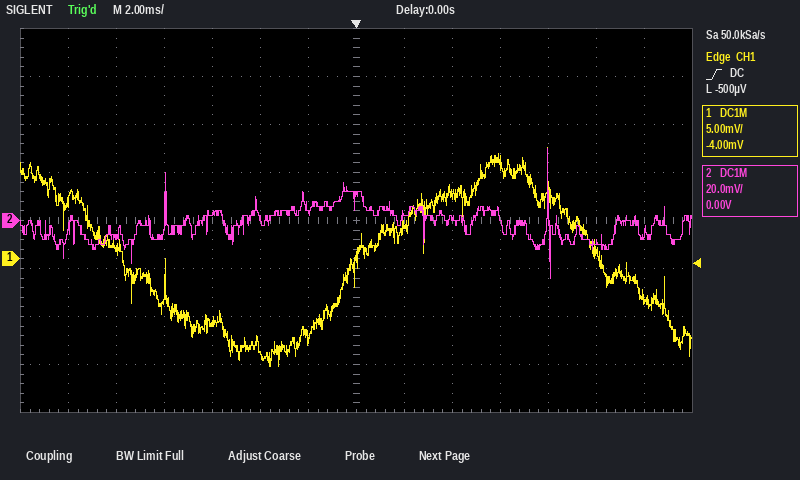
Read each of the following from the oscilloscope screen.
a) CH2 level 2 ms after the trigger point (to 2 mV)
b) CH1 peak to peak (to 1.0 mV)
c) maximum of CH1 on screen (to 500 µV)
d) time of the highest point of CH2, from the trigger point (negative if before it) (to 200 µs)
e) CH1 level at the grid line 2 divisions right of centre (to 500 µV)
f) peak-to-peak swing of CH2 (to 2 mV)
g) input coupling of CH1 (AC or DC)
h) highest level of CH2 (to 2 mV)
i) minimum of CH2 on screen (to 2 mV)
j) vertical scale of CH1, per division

2 mV
23.0 mV
11.5 mV
+8.0 ms
6.5 mV
54 mV
DC
30 mV
-24 mV
5 mV
